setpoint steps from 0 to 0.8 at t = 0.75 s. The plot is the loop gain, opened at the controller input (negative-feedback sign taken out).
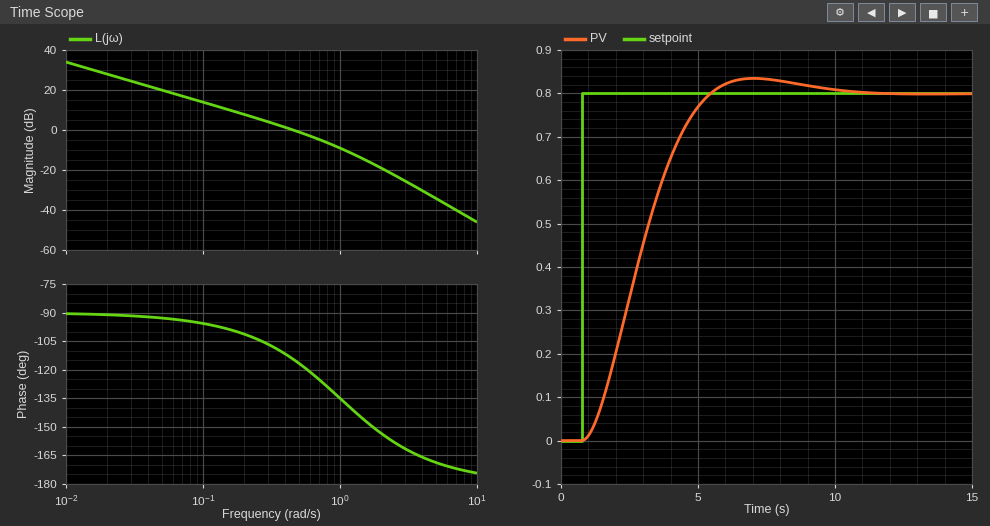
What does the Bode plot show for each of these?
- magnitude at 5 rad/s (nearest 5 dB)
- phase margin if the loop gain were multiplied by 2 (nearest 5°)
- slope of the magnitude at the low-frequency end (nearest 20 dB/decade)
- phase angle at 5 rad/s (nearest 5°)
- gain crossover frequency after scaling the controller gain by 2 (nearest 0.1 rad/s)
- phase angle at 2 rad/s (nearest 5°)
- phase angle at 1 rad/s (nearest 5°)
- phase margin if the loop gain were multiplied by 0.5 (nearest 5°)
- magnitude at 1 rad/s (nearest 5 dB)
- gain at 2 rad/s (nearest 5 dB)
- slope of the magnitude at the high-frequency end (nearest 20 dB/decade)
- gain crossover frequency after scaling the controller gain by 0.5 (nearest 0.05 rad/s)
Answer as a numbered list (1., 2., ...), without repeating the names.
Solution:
1. -35 dB
2. 50°
3. -20 dB/decade
4. -170°
5. 0.8 rad/s
6. -155°
7. -135°
8. 75°
9. -10 dB
10. -20 dB
11. -40 dB/decade
12. 0.25 rad/s
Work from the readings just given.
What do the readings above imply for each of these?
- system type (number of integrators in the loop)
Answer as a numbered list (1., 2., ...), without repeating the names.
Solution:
1. 1
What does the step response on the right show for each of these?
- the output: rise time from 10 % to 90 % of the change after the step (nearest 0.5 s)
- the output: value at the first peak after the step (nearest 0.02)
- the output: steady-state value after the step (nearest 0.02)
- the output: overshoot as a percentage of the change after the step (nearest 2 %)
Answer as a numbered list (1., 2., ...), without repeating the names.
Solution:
1. 3.0 s
2. 0.84
3. 0.80
4. 4 %
